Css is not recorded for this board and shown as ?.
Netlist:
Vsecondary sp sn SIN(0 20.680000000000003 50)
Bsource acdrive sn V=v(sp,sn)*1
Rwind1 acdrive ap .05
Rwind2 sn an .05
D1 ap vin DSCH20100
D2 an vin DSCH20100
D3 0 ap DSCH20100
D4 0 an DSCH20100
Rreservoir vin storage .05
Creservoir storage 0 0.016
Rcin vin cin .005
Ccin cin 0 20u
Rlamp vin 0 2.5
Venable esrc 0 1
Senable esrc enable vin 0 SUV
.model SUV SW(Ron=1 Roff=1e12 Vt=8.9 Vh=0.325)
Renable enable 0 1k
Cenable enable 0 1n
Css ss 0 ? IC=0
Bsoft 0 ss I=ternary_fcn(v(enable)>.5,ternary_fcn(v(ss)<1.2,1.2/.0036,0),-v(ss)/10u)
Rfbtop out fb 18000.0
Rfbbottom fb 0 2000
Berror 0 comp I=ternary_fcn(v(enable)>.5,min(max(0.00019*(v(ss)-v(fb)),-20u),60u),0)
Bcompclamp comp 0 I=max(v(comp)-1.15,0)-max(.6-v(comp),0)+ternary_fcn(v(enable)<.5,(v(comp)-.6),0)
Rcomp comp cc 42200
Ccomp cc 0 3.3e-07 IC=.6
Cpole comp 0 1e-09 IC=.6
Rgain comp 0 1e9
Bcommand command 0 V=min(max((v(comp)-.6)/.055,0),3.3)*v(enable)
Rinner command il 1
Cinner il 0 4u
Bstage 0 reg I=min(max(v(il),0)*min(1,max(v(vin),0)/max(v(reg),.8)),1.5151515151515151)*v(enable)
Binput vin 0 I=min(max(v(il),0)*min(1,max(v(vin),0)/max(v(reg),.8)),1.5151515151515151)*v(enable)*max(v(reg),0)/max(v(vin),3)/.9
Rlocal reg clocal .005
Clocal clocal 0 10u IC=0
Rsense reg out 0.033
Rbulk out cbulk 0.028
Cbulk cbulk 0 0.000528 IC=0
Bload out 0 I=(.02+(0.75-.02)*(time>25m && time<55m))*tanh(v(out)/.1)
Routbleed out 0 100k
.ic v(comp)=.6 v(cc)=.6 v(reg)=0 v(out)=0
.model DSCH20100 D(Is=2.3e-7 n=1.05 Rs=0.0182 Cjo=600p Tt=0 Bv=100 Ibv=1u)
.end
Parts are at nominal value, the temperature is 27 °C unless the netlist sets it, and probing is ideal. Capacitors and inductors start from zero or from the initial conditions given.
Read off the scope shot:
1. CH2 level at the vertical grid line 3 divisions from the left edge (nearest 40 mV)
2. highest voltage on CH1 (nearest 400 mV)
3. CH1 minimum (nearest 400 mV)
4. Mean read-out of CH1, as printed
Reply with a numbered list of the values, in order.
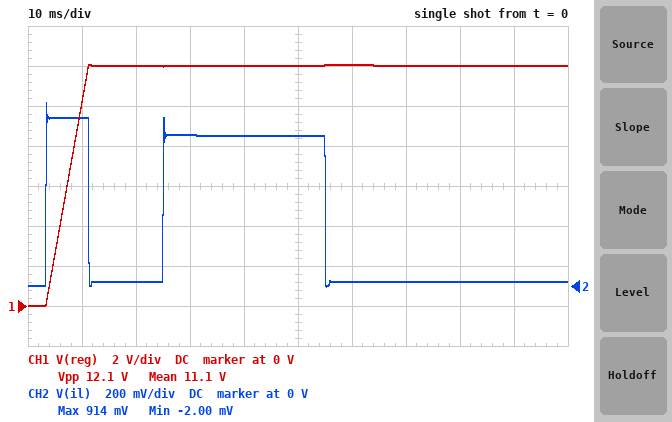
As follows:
1. 760 mV
2. 12.0 V
3. 0 V
4. 11.1 V
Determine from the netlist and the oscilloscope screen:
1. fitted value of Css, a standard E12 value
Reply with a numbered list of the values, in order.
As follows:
1. 2.2 F
